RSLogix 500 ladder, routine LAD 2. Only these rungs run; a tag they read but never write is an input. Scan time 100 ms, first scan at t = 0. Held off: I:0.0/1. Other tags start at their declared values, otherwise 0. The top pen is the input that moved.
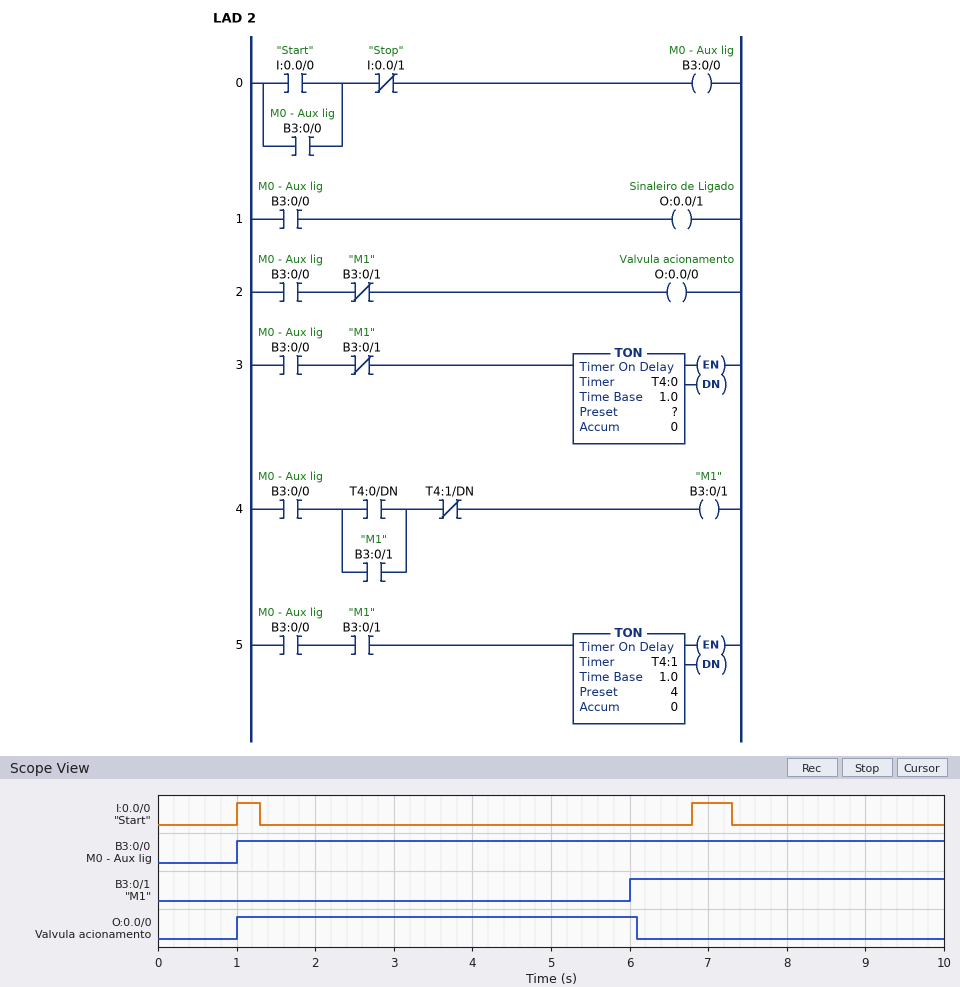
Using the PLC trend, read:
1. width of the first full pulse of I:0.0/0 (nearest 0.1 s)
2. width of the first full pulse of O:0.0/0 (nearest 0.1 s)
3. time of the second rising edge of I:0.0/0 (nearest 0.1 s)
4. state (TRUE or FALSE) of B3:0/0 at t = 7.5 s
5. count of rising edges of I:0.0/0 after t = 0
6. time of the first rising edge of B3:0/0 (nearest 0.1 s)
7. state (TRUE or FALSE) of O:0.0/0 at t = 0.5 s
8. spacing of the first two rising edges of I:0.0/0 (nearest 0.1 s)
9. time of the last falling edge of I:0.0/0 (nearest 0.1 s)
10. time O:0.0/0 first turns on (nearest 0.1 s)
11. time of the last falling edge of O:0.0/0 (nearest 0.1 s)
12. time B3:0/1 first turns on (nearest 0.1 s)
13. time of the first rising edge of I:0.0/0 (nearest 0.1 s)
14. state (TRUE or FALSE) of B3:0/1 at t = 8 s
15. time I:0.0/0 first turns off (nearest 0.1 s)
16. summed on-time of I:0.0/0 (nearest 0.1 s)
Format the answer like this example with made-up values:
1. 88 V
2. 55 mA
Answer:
1. 0.3 s
2. 5.1 s
3. 6.8 s
4. TRUE
5. 2
6. 1.0 s
7. FALSE
8. 5.8 s
9. 7.3 s
10. 1.0 s
11. 6.1 s
12. 6.0 s
13. 1.0 s
14. TRUE
15. 1.3 s
16. 0.8 s
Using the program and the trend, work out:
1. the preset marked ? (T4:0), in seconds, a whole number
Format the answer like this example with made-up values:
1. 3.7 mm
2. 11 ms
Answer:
1. 5 s
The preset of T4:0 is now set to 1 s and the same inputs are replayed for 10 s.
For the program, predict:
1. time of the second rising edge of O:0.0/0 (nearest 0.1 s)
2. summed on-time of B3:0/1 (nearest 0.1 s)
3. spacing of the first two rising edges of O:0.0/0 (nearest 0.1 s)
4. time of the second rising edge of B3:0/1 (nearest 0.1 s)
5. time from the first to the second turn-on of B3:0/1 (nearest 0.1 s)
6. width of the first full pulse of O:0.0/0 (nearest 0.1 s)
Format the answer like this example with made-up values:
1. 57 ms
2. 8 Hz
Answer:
1. 6.2 s
2. 6.9 s
3. 5.2 s
4. 7.2 s
5. 5.2 s
6. 1.1 s
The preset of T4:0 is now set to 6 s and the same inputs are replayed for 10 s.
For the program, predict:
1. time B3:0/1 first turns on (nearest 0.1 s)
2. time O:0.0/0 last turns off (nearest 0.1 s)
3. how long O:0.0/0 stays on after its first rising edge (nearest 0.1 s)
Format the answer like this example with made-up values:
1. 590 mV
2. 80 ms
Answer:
1. 7.0 s
2. 7.1 s
3. 6.1 s
